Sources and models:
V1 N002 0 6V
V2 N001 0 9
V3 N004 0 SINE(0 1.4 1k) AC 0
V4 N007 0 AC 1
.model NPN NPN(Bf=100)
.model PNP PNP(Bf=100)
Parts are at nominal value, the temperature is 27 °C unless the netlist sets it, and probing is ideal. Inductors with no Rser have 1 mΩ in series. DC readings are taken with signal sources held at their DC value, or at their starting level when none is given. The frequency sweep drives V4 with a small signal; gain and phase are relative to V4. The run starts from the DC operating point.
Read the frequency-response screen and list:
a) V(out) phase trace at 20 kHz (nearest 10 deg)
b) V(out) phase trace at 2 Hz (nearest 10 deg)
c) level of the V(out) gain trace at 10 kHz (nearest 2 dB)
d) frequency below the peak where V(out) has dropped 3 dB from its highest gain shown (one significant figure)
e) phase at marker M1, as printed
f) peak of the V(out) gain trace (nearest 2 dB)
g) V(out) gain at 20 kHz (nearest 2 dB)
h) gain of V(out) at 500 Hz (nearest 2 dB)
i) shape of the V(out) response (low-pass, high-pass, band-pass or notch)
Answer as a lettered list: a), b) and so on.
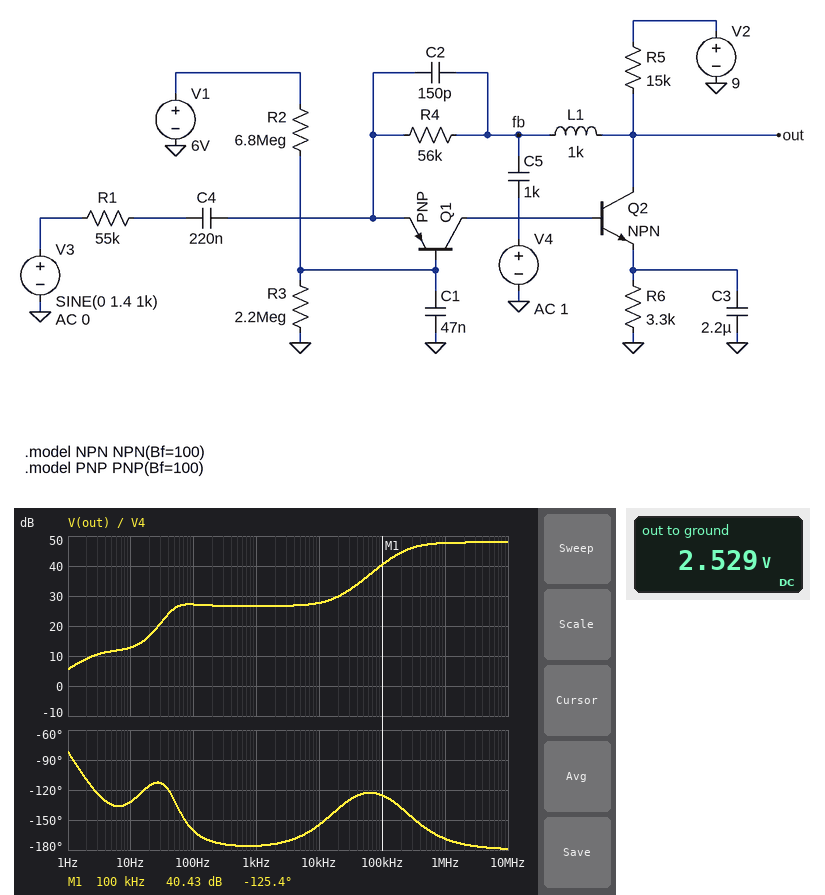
a) -140 deg
b) -110 deg
c) 28 dB
d) 200 kHz
e) -125.4 deg
f) 48 dB
g) 30 dB
h) 26 dB
i) high-pass
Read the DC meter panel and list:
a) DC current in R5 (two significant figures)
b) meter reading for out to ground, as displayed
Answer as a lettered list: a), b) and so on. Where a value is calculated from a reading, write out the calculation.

a) (9 V - 2.529 V) / 15 kΩ = 430 µA
b) 2.529 V
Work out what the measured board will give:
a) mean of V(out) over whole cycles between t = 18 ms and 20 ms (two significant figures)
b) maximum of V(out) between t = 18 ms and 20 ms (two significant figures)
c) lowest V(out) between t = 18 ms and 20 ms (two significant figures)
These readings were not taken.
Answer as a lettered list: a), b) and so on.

a) 4.6 V
b) 8.3 V
c) 980 mV
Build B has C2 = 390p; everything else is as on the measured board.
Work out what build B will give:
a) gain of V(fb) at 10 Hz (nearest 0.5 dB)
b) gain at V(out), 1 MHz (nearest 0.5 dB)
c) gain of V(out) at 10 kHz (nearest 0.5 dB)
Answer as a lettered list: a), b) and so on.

a) 0 dB
b) 48.0 dB
c) 31.0 dB
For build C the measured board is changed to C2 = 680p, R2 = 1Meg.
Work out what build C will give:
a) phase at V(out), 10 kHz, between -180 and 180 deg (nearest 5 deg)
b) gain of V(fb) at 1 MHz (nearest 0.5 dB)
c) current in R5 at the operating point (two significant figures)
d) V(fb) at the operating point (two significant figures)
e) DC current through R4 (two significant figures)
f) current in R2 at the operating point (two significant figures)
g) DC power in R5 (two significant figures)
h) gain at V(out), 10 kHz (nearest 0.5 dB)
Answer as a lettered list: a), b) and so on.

a) -130 deg
b) 0 dB
c) 270 µA
d) 4.9 V
e) 2.7 µA
f) 1.9 µA
g) 1.1 mW
h) 34.0 dB
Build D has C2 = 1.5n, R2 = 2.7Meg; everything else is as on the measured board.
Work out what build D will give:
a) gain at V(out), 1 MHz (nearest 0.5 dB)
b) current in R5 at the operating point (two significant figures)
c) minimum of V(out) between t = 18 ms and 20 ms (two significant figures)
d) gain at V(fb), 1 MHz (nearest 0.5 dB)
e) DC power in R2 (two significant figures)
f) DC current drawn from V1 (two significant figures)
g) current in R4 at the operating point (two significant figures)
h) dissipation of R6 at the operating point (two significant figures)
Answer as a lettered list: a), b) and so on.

a) 46.5 dB
b) 360 µA
c) 930 mV
d) 0 dB
e) 3.9 µW
f) 1.2 µA
g) 3.6 µA
h) 430 µW
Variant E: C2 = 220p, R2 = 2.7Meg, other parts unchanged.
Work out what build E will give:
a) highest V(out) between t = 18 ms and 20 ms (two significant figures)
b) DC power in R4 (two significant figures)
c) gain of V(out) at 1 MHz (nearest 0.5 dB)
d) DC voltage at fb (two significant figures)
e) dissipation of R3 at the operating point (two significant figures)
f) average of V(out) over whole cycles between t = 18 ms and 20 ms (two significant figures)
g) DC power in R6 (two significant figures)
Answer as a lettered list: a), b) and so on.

a) 8.6 V
b) 730 nW
c) 46.5 dB
d) 3.6 V
e) 3.4 µW
f) 4.9 V
g) 430 µW
